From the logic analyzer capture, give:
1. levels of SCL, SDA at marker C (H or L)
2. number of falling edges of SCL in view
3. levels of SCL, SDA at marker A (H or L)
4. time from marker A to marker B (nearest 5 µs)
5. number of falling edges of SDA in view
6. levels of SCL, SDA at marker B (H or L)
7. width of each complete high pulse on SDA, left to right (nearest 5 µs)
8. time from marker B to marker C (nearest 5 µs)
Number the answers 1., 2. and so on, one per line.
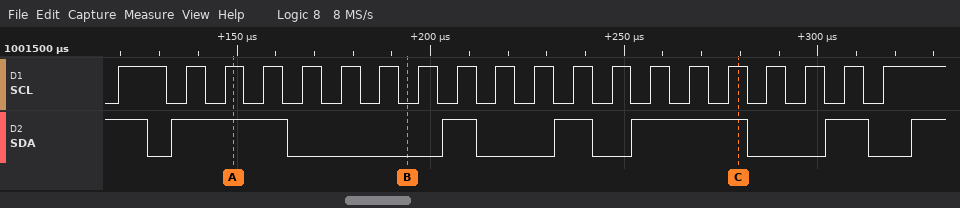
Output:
1. SCL=H, SDA=H
2. 19
3. SCL=H, SDA=H
4. 45 µs
5. 6
6. SCL=L, SDA=L
7. 30 µs, 10 µs, 10 µs, 30 µs, 10 µs
8. 85 µs
